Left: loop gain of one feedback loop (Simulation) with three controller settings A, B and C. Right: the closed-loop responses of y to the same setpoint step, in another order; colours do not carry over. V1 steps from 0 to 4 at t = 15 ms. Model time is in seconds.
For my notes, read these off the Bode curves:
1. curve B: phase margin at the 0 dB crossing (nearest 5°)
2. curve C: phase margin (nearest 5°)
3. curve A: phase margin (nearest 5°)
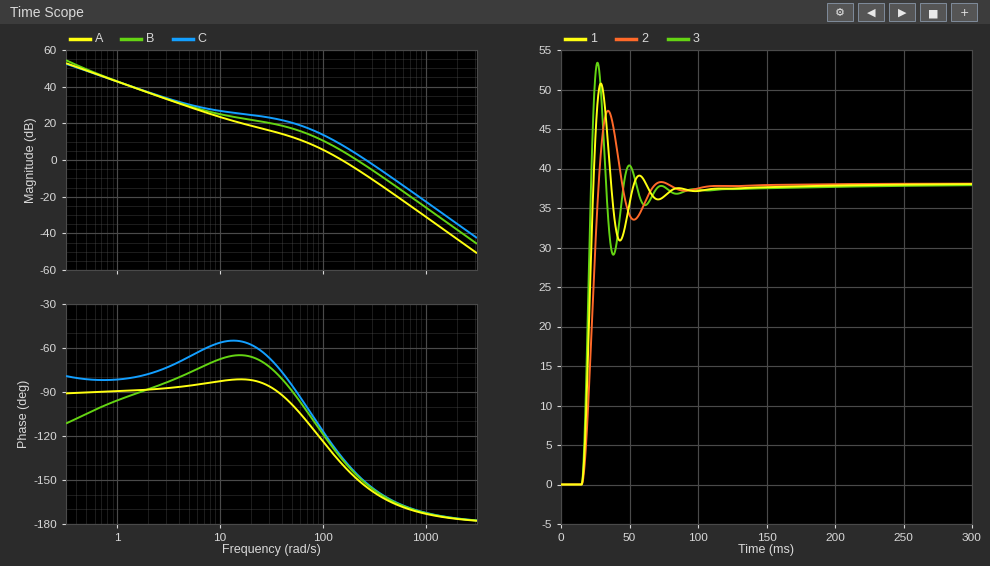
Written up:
35°
30°
40°
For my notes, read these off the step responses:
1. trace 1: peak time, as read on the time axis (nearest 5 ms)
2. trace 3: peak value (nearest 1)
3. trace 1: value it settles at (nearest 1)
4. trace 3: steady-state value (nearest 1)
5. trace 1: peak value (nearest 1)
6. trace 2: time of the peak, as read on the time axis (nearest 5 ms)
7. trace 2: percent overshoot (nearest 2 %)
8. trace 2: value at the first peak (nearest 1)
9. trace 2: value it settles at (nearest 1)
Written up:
30 ms
53
38
38
51
35 ms
24 %
47
38
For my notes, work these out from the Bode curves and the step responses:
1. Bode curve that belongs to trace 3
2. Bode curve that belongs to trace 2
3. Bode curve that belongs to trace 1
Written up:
C
A
B
